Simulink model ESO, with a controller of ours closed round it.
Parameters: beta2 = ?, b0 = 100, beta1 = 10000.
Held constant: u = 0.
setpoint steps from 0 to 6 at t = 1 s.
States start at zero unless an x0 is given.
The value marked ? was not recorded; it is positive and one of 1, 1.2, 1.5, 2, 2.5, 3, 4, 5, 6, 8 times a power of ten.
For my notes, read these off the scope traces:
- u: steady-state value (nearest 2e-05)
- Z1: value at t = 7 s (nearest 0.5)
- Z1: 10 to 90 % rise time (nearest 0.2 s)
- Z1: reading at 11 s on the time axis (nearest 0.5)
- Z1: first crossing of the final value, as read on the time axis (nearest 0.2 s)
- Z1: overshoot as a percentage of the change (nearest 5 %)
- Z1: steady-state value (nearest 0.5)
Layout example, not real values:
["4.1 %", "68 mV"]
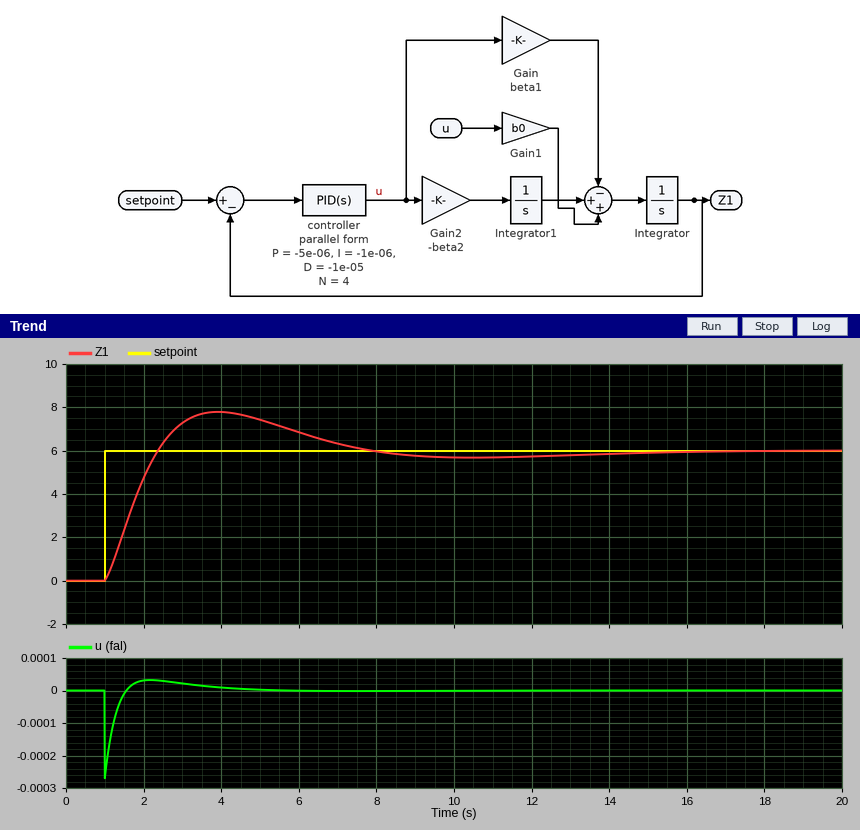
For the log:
["0.00000", "6.5", "1.0 s", "5.5", "2.4 s", "30 %", "6.0"]
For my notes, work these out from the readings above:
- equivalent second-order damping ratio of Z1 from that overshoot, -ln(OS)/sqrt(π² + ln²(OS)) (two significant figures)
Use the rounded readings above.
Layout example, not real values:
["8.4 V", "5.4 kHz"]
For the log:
["0.36"]
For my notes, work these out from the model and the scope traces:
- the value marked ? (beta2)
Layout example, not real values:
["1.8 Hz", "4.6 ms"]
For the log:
["100000"]
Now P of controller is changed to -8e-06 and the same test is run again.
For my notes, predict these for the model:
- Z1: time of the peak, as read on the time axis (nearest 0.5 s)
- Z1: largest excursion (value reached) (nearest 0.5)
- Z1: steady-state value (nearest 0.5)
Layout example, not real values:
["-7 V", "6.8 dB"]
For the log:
["3.5 s", "8.0", "6.0"]
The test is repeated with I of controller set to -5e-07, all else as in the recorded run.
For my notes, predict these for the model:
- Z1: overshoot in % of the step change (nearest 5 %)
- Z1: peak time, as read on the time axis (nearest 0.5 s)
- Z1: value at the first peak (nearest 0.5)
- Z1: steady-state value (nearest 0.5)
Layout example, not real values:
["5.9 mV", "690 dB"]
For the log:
["25 %", "4.0 s", "7.5", "6.0"]
